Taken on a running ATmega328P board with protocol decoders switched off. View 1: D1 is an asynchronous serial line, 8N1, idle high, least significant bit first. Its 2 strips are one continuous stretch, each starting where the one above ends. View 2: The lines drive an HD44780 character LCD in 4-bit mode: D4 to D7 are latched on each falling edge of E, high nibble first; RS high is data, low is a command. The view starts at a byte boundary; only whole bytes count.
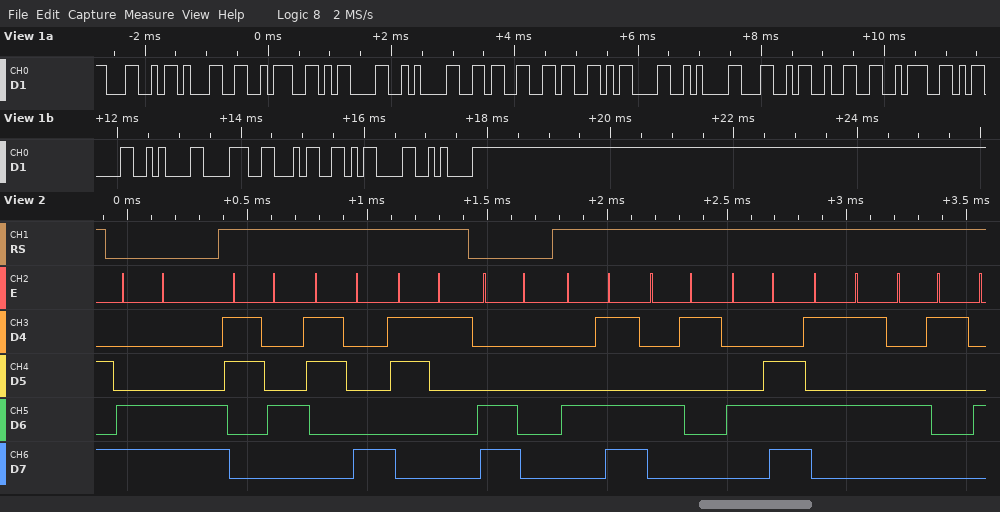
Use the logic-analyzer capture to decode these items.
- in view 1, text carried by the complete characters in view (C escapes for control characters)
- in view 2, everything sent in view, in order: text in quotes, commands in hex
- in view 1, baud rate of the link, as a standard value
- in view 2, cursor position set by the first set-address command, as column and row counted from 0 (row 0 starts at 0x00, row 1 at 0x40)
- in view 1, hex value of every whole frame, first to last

"L1:\r\n66\r\nL2:\r\n84\r\n"
0xCC "481" 0xC0 "MANUA"
9600 baud
column 12, row 1
4C 31 3A 0D 0A 36 36 0D 0A 4C 32 3A 0D 0A 38 34 0D 0A
